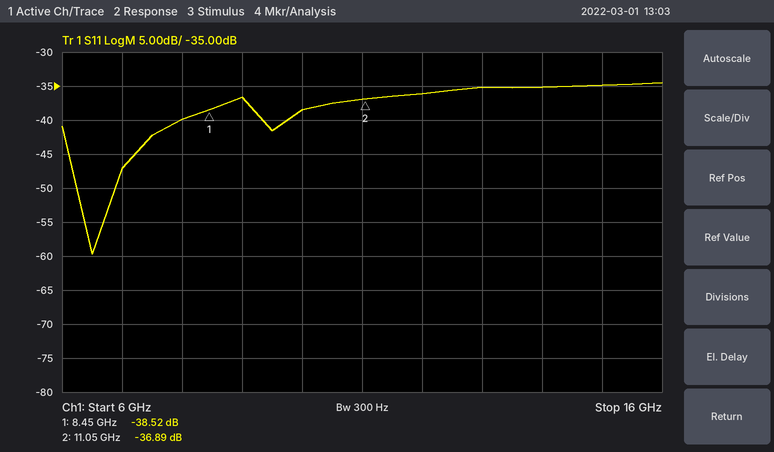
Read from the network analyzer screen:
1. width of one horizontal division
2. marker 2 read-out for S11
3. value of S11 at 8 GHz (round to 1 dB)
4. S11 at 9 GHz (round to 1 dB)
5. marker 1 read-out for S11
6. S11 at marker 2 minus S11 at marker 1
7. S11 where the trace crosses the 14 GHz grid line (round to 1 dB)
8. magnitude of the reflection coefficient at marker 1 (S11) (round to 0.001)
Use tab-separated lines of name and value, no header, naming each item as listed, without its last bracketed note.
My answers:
width of one horizontal division	1 GHz
marker 2 read-out for S11	-36.89 dB
value of S11 at 8 GHz	-40 dB
S11 at 9 GHz	-37 dB
marker 1 read-out for S11	-38.52 dB
S11 at marker 2 minus S11 at marker 1	1.63 dB
S11 where the trace crosses the 14 GHz grid line	-35 dB
magnitude of the reflection coefficient at marker 1 (S11)	0.012
